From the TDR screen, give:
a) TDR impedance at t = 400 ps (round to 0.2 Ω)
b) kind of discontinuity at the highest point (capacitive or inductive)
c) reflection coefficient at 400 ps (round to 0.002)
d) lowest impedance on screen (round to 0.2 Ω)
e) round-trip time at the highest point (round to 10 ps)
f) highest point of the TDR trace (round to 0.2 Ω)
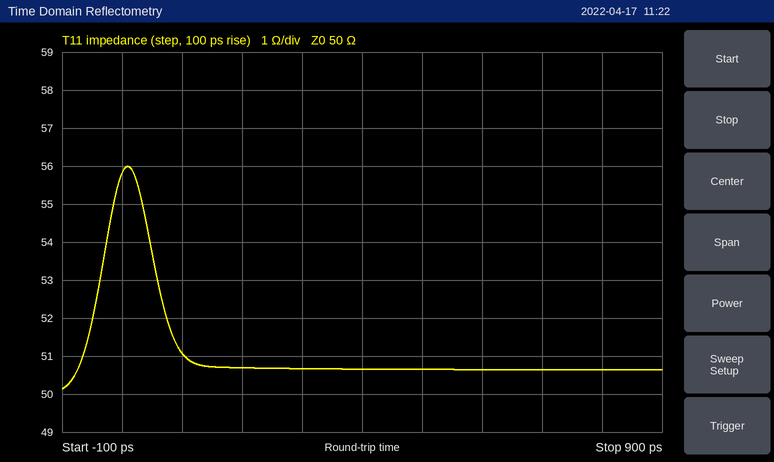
50.6 Ω
inductive
+0.006
50.2 Ω
10 ps
56.0 Ω
